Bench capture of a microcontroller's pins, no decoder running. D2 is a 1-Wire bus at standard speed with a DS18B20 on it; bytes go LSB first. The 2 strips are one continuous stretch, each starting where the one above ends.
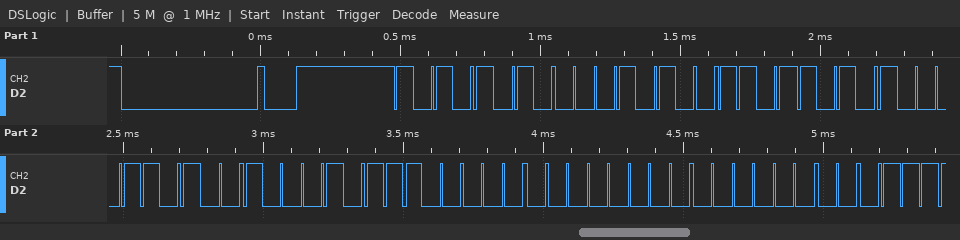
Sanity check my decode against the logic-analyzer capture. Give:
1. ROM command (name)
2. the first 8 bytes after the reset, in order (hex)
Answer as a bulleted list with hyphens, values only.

- Match ROM
- 55 28 5B B1 44 07 00 00
